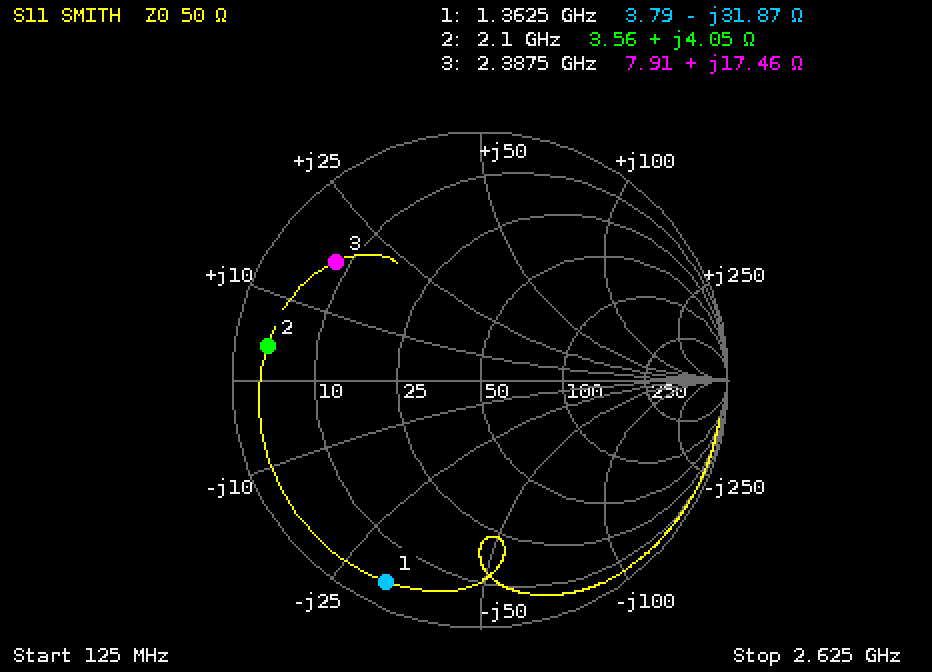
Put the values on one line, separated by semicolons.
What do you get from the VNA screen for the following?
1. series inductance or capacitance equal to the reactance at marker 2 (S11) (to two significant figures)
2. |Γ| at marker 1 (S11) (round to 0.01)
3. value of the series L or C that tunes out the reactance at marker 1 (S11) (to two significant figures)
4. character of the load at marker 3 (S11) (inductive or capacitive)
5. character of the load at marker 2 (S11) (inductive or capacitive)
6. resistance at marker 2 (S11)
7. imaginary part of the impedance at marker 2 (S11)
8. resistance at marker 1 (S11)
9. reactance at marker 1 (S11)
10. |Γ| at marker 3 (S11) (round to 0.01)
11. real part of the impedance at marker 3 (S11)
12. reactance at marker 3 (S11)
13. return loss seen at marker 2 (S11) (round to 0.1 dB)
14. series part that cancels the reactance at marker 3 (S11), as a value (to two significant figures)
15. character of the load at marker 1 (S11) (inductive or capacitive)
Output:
310 pH; 0.90; 3.7 nH; inductive; inductive; 3.56 Ω; +4.05 Ω; 3.79 Ω; -31.87 Ω; 0.75; 7.91 Ω; +17.46 Ω; 1.2 dB; 3.8 pF; capacitive
